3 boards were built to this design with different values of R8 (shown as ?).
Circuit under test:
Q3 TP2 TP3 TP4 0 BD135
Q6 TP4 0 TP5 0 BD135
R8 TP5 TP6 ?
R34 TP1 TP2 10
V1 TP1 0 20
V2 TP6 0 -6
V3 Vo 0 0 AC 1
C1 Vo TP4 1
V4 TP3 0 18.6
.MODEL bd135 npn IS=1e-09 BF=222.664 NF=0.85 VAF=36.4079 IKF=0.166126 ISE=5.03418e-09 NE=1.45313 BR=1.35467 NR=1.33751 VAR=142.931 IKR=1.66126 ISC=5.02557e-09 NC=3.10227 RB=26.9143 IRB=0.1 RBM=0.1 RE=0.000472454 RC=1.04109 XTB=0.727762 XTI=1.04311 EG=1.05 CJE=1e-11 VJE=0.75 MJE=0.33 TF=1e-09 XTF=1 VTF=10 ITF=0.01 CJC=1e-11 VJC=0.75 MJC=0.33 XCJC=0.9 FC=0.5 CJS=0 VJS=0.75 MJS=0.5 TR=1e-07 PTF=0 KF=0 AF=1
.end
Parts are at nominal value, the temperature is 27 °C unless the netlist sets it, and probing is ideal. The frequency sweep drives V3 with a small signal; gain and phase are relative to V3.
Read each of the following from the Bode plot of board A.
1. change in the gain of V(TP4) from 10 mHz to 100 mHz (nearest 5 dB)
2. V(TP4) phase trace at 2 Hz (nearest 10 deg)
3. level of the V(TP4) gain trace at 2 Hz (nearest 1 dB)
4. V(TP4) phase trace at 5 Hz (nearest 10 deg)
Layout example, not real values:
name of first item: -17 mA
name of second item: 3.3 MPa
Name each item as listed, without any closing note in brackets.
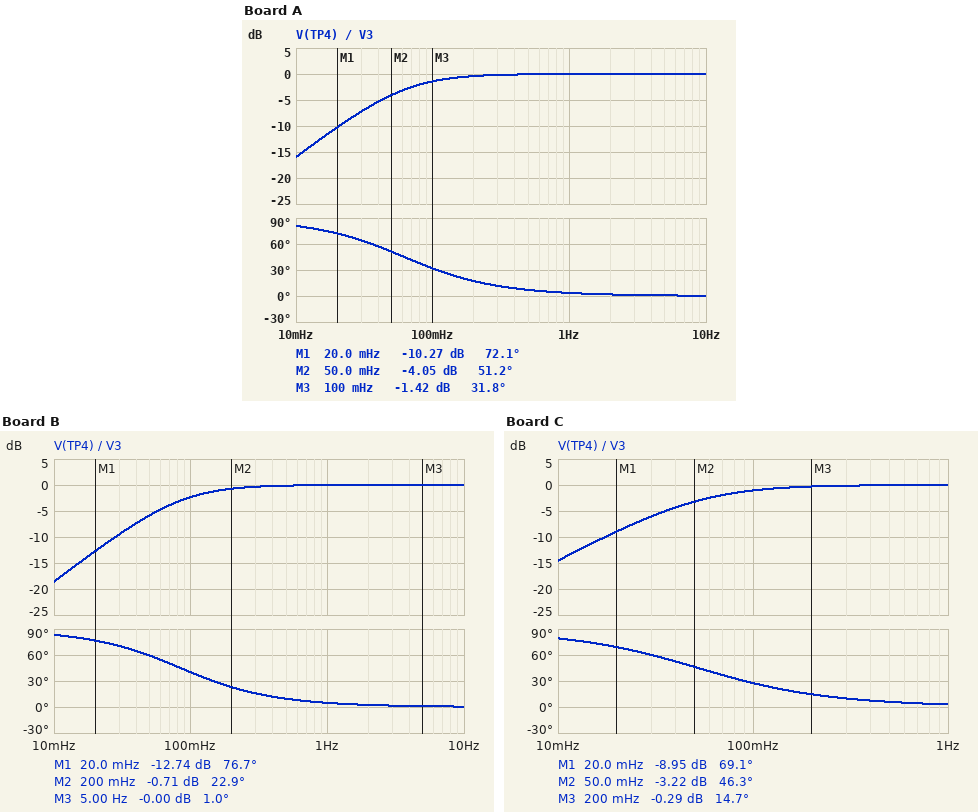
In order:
change in the gain of V(TP4) from 10 mHz to 100 mHz: 15 dB
V(TP4) phase trace at 2 Hz: 0 deg
level of the V(TP4) gain trace at 2 Hz: 0 dB
V(TP4) phase trace at 5 Hz: 0 deg
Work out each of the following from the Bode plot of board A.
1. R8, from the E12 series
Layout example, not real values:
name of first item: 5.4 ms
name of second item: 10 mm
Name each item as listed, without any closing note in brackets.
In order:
R8, from the E12 series: 560 Ω
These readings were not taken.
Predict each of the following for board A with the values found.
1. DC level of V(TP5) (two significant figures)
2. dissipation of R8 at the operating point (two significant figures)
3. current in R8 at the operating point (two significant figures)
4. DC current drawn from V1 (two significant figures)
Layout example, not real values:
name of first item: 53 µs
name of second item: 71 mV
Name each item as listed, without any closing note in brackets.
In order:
DC level of V(TP5): -350 mV
dissipation of R8 at the operating point: 57 mW
current in R8 at the operating point: 10 mA
DC current drawn from V1: 9.9 mA
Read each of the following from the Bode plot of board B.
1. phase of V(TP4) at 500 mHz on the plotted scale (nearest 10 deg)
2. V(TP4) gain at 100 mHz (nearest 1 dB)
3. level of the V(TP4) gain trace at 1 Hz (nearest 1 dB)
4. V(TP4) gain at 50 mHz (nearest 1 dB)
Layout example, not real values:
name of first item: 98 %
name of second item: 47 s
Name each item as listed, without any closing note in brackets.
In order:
phase of V(TP4) at 500 mHz on the plotted scale: 10 deg
V(TP4) gain at 100 mHz: -2 dB
level of the V(TP4) gain trace at 1 Hz: 0 dB
V(TP4) gain at 50 mHz: -6 dB
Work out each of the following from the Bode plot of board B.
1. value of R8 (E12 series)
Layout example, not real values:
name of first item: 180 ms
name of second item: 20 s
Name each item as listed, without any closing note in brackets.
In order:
value of R8: 390 Ω
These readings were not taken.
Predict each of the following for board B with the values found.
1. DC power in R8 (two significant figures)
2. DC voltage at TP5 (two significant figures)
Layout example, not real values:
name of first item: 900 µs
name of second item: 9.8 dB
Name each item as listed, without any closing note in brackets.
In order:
DC power in R8: 82 mW
DC voltage at TP5: -360 mV
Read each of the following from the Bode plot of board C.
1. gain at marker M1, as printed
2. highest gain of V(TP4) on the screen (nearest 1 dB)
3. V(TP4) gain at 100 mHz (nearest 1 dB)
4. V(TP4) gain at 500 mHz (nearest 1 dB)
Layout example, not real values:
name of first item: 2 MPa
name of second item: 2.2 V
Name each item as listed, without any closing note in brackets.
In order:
gain at marker M1, as printed: -8.95 dB
highest gain of V(TP4) on the screen: 0 dB
V(TP4) gain at 100 mHz: -1 dB
V(TP4) gain at 500 mHz: 0 dB
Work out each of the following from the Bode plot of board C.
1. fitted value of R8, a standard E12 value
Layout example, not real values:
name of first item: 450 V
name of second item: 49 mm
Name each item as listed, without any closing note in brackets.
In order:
fitted value of R8, a standard E12 value: 680 Ω
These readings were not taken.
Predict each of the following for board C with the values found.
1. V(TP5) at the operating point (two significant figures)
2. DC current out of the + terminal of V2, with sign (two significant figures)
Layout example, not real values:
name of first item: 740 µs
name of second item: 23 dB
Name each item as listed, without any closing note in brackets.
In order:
V(TP5) at the operating point: -340 mV
DC current out of the + terminal of V2, with sign: -8.3 mA
